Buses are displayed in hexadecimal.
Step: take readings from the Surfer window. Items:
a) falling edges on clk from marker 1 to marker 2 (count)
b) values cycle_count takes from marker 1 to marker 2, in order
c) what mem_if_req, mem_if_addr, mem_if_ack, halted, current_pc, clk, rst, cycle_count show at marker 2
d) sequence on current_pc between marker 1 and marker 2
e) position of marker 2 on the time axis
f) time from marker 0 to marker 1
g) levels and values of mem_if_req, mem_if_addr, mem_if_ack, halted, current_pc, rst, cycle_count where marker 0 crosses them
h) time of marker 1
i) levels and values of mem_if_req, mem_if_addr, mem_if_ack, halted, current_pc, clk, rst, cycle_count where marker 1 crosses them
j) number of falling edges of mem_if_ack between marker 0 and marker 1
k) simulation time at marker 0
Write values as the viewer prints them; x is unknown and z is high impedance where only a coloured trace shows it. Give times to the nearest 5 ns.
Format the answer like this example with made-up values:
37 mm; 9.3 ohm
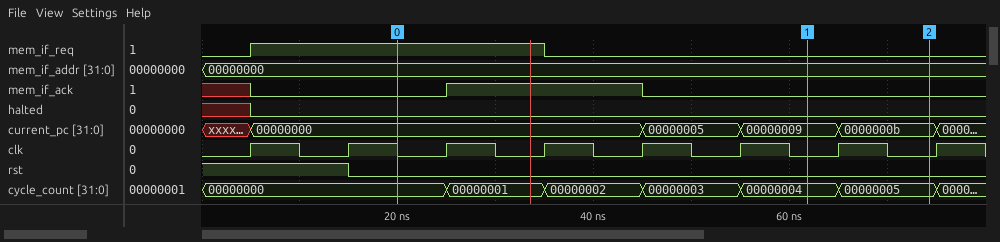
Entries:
1; 00000004, 00000005; mem_if_req=0, mem_if_addr=00000000, mem_if_ack=0, halted=0, current_pc=0000000b, clk=0, rst=0, cycle_count=00000005; 00000009, 0000000b; 75 ns; 40 ns; mem_if_req=1, mem_if_addr=00000000, mem_if_ack=0, halted=0, current_pc=00000000, rst=0, cycle_count=00000000; 60 ns; mem_if_req=0, mem_if_addr=00000000, mem_if_ack=0, halted=0, current_pc=00000009, clk=0, rst=0, cycle_count=00000004; 1; 20 ns
